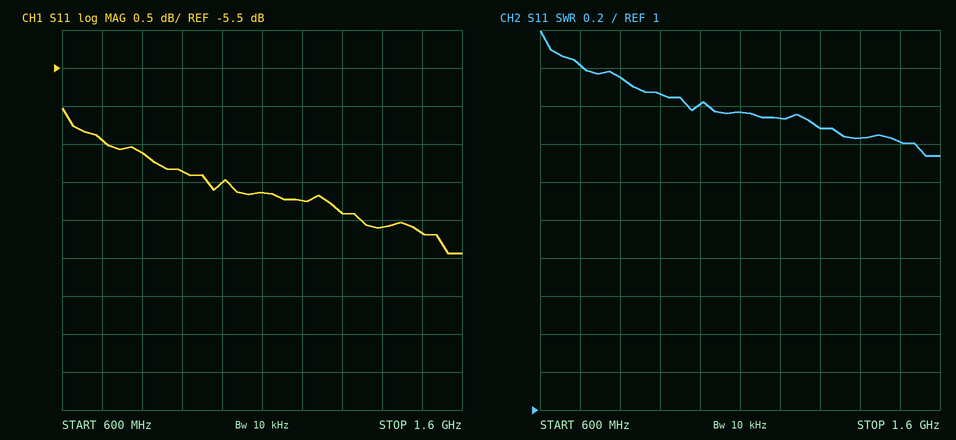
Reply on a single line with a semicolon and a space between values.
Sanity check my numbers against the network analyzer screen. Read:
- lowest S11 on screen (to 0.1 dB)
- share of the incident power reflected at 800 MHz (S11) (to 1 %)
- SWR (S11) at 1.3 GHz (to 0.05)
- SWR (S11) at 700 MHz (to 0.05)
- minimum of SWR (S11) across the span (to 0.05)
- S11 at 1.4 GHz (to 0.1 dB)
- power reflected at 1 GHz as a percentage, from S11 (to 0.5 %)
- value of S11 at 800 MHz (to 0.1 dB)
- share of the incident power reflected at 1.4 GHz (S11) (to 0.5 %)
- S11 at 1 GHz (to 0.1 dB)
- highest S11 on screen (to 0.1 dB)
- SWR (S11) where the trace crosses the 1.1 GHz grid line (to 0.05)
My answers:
-7.9 dB; 22 %; 2.50; 2.80; 2.35; -7.6 dB; 20.0 %; -6.6 dB; 17.5 %; -7.0 dB; -6.0 dB; 2.55
